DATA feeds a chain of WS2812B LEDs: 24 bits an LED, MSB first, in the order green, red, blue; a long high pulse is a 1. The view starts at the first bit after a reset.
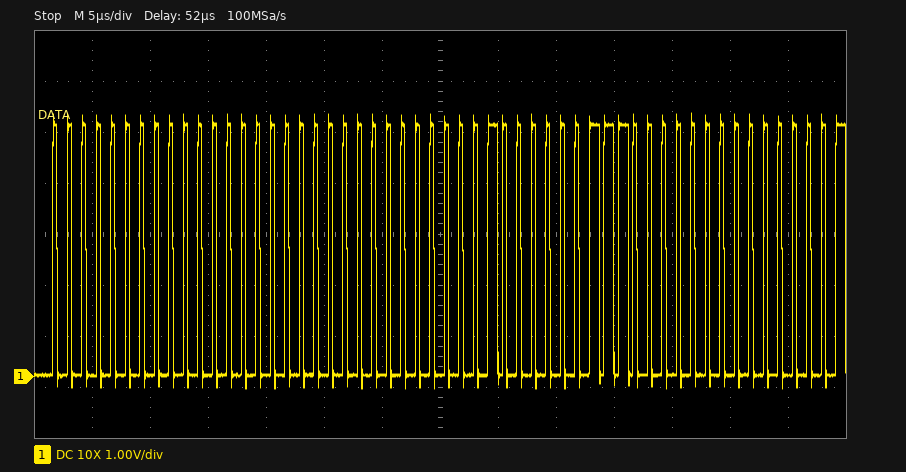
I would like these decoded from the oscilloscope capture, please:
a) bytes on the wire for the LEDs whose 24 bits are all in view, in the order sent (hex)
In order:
00 00 00 02 07 00
